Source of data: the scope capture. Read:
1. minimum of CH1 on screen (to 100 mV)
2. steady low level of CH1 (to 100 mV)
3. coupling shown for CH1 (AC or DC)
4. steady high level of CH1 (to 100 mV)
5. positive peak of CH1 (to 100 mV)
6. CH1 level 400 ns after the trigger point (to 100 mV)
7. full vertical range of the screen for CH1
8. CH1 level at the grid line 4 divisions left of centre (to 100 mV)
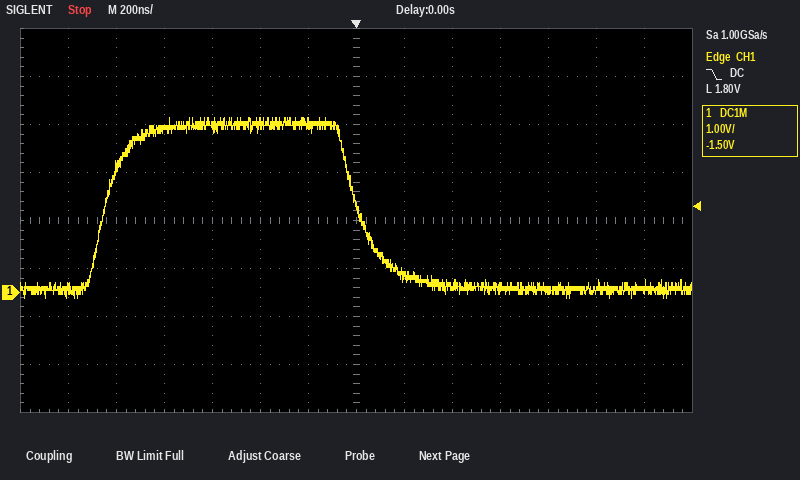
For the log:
-100 mV
100 mV
DC
3.5 V
3.6 V
100 mV
8 V
3.4 V
